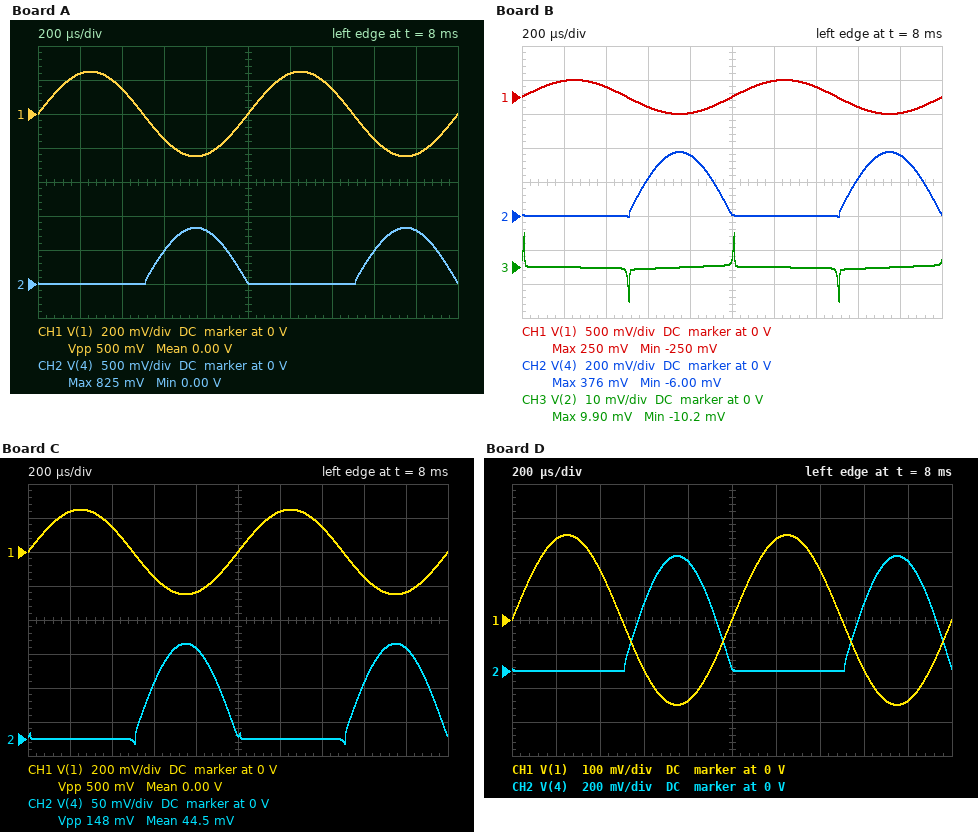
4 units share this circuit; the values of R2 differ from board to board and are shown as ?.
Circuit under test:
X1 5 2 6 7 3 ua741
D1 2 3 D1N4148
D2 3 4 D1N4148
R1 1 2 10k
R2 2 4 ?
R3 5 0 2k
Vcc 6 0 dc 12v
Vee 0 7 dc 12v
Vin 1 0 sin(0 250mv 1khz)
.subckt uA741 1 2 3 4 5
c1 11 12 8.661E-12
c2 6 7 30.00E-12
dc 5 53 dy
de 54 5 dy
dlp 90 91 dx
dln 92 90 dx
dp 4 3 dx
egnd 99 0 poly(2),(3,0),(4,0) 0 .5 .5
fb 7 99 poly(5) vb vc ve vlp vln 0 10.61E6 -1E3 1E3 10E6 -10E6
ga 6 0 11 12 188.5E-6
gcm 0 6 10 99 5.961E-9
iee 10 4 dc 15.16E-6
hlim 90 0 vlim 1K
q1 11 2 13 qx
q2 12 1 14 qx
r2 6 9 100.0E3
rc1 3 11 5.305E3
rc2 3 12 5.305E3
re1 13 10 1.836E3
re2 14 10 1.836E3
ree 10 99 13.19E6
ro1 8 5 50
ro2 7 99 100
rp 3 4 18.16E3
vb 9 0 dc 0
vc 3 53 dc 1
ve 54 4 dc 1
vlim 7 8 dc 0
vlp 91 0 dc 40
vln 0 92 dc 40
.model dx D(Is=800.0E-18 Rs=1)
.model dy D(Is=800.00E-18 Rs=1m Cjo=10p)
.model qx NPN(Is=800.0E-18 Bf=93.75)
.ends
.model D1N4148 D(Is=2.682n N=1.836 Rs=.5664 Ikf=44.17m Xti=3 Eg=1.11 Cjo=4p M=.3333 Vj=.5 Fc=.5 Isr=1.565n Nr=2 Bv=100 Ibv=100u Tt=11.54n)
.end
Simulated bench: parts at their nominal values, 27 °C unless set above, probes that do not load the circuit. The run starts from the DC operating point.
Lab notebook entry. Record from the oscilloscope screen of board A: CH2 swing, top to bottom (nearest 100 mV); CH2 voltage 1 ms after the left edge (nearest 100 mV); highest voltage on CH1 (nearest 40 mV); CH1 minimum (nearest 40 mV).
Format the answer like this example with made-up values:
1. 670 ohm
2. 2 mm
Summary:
1. 800 mV
2. 0 V
3. 240 mV
4. -240 mV
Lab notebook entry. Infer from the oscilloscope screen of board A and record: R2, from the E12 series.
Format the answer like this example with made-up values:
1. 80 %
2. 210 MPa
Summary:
1. 33 kΩ
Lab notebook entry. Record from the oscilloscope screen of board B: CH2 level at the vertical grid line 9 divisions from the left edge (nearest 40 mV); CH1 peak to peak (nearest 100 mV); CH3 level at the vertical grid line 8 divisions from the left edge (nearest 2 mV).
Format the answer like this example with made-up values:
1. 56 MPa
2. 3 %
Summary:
1. 360 mV
2. 500 mV
3. 0 V
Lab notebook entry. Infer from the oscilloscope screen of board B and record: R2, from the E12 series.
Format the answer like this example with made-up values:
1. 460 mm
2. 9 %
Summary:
1. 15 kΩ
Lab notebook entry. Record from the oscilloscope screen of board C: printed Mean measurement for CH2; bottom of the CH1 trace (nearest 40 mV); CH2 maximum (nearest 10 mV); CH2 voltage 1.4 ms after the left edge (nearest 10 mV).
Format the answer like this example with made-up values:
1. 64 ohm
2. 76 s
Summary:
1. 44.5 mV
2. -240 mV
3. 140 mV
4. 0 V
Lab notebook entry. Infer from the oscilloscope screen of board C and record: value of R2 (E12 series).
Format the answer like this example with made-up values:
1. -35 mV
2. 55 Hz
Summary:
1. 5.6 kΩ
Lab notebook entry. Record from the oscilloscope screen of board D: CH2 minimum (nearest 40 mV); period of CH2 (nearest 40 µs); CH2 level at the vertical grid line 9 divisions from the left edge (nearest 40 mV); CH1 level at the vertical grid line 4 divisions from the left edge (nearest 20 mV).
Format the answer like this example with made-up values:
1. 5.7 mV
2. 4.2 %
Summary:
1. 0 V
2. 1.00 ms
3. 640 mV
4. -240 mV
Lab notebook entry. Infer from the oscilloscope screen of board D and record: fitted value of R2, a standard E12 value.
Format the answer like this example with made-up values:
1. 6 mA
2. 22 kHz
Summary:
1. 27 kΩ
